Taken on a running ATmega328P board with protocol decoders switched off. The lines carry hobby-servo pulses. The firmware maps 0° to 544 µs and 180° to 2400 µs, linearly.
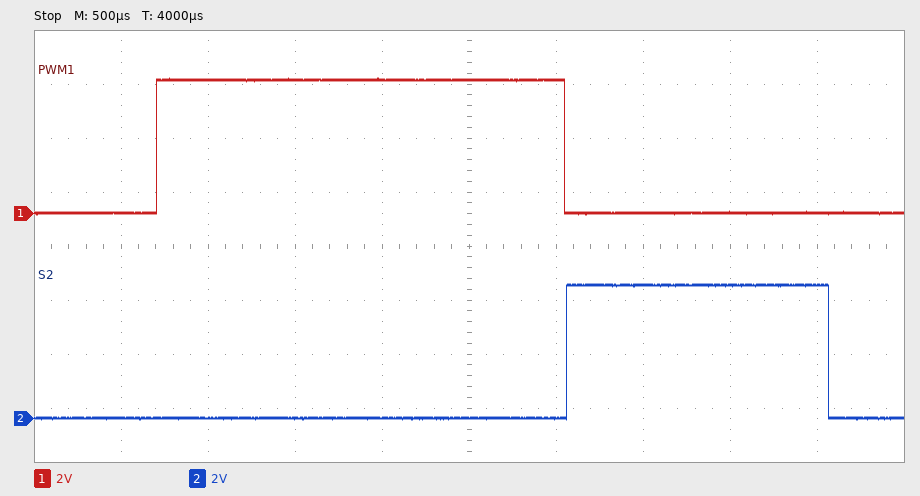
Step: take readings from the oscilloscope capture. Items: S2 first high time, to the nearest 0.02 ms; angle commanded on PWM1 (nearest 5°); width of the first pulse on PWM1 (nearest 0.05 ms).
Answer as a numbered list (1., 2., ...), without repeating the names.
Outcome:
1. 1.50 ms
2. 175°
3. 2.35 ms
